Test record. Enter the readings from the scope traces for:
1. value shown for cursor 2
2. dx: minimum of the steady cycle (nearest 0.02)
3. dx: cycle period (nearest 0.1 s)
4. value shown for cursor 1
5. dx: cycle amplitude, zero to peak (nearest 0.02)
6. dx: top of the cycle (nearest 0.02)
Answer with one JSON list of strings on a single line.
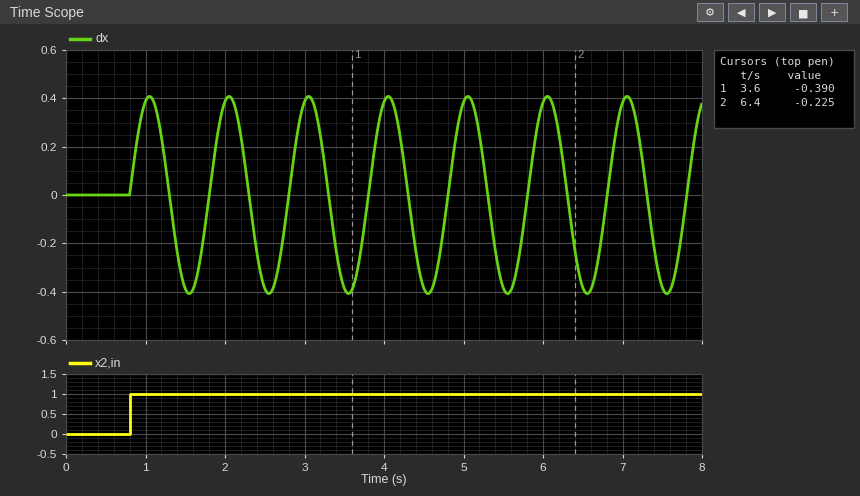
["-0.225", "-0.40", "1.0 s", "-0.390", "0.40", "0.40"]
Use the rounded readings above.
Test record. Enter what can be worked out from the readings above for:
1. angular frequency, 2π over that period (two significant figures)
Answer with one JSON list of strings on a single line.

["6.3 rad/s"]
